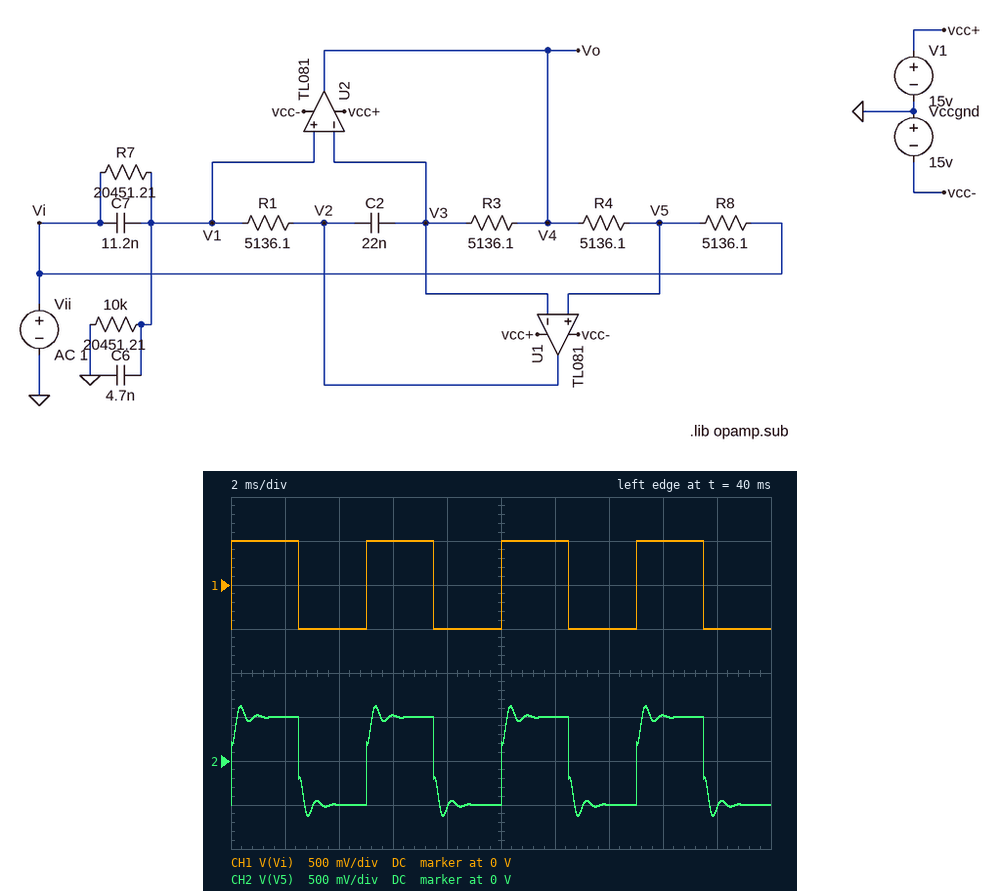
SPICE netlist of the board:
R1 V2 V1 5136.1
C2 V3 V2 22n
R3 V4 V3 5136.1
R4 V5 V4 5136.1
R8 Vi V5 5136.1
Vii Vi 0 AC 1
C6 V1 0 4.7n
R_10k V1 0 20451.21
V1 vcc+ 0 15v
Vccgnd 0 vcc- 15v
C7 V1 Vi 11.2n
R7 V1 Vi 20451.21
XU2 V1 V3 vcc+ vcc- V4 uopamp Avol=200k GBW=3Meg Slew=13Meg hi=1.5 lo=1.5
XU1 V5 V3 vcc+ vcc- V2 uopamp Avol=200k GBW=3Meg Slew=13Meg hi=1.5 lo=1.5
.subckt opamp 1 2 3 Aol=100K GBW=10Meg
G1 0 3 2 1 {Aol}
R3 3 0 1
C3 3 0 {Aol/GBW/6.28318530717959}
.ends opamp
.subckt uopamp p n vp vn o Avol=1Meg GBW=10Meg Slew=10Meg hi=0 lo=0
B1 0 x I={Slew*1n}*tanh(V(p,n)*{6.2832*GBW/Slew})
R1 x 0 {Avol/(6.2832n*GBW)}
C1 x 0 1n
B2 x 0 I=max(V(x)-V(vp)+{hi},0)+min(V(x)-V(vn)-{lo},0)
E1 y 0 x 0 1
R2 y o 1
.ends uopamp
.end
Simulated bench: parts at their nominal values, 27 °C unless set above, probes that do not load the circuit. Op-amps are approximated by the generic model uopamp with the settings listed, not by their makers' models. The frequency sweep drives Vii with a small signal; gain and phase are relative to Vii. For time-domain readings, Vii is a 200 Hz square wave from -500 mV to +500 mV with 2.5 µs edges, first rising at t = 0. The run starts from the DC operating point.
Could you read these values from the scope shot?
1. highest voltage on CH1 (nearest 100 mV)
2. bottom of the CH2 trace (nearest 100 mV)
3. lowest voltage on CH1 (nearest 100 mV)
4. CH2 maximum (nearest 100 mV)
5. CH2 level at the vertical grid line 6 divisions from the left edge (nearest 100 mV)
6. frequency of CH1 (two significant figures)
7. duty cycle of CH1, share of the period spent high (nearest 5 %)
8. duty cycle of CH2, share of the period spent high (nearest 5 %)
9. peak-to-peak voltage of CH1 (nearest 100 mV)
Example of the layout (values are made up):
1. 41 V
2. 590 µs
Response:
1. 500 mV
2. -600 mV
3. -500 mV
4. 600 mV
5. 500 mV
6. 200 Hz
7. 50 %
8. 50 %
9. 1.0 V
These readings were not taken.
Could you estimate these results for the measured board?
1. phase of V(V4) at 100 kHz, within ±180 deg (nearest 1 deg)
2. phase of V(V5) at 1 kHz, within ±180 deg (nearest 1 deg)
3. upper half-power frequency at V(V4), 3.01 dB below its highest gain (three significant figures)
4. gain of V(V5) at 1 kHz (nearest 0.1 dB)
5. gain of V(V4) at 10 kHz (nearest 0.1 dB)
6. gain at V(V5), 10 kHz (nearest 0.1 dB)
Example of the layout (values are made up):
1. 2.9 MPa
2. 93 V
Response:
1. 3 deg
2. -16 deg
3. 1.73 kHz
4. 0.4 dB
5. -8.2 dB
6. -3.2 dB
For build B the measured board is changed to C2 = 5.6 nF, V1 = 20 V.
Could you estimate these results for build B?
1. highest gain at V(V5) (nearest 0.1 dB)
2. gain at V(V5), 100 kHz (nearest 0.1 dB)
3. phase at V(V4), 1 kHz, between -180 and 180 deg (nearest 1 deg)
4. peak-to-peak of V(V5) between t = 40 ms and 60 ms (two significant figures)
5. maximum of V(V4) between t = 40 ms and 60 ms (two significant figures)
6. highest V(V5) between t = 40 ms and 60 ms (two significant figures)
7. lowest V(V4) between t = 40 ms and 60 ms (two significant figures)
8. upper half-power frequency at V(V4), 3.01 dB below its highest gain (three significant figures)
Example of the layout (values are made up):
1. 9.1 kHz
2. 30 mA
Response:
1. 2.7 dB
2. -3.0 dB
3. -6 deg
4. 1.4 V
5. 880 mV
6. 690 mV
7. -880 mV
8. 3.52 kHz
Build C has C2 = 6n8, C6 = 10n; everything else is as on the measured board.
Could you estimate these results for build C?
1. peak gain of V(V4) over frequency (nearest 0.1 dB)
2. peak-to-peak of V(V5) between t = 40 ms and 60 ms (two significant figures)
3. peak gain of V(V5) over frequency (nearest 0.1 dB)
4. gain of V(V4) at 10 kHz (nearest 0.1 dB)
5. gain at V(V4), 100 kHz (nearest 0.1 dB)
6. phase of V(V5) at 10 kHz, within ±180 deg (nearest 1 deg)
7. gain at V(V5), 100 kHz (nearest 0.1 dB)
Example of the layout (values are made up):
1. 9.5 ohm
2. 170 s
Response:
1. 10.5 dB
2. 1.6 V
3. 5.5 dB
4. -40.5 dB
5. -23.4 dB
6. 0 deg
7. -5.5 dB
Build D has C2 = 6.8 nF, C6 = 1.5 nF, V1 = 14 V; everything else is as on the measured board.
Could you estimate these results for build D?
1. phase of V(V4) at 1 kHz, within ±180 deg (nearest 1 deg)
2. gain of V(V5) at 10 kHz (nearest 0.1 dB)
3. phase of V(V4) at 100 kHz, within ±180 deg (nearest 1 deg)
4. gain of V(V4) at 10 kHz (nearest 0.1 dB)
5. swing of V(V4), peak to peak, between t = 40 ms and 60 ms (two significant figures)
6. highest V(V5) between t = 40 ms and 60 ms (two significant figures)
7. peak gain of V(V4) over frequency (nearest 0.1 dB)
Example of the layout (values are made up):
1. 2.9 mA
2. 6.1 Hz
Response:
1. -7 deg
2. -1.3 dB
3. 1 deg
4. -2.8 dB
5. 1.4 V
6. 600 mV
7. 0.9 dB
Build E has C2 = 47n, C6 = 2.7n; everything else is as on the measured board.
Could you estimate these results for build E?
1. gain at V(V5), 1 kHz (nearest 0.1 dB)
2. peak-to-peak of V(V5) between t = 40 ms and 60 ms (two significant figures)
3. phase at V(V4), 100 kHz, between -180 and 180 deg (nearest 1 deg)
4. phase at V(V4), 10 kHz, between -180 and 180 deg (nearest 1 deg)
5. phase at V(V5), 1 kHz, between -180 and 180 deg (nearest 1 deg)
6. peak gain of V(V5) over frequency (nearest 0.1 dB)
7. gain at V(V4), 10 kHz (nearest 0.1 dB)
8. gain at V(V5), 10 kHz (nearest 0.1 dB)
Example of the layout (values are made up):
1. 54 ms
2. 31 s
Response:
1. -2.9 dB
2. 1.1 V
3. 2 deg
4. 7 deg
5. -27 deg
6. 0 dB
7. -4.4 dB
8. -1.9 dB
